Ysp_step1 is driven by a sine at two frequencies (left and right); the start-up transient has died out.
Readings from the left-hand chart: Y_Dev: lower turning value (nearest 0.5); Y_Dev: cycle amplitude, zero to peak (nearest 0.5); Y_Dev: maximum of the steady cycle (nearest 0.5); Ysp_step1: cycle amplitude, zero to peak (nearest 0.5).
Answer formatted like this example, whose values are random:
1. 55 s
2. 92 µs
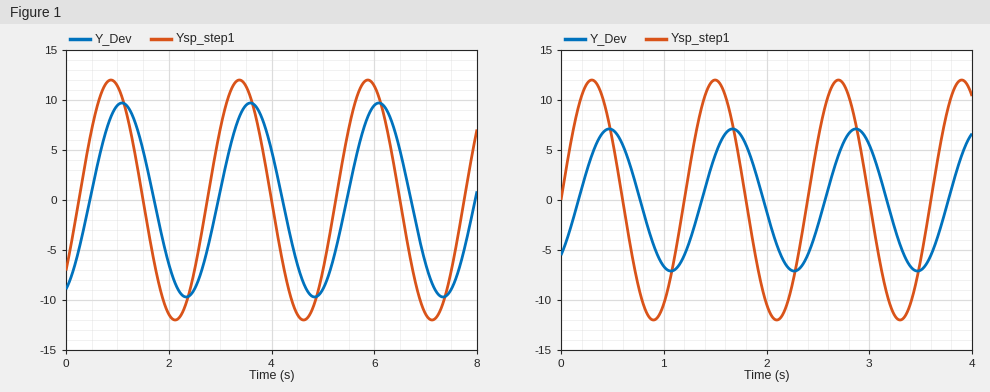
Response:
1. -9.5
2. 9.5
3. 9.5
4. 12.0
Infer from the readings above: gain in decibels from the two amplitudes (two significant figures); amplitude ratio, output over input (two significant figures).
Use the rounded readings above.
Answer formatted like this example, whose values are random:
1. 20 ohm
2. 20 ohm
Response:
1. -2.0 dB
2. 0.79
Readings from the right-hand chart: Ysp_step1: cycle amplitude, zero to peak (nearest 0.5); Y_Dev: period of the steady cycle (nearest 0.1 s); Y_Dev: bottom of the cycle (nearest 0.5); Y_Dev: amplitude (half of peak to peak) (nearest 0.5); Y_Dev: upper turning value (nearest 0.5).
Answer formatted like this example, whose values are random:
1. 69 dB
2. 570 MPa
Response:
1. 12.0
2. 1.2 s
3. -7.0
4. 7.0
5. 7.0
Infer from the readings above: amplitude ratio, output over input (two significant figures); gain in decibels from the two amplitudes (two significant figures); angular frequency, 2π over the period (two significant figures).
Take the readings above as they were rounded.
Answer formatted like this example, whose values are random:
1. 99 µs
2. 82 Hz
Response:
1. 0.58
2. -4.7 dB
3. 5.2 rad/s
